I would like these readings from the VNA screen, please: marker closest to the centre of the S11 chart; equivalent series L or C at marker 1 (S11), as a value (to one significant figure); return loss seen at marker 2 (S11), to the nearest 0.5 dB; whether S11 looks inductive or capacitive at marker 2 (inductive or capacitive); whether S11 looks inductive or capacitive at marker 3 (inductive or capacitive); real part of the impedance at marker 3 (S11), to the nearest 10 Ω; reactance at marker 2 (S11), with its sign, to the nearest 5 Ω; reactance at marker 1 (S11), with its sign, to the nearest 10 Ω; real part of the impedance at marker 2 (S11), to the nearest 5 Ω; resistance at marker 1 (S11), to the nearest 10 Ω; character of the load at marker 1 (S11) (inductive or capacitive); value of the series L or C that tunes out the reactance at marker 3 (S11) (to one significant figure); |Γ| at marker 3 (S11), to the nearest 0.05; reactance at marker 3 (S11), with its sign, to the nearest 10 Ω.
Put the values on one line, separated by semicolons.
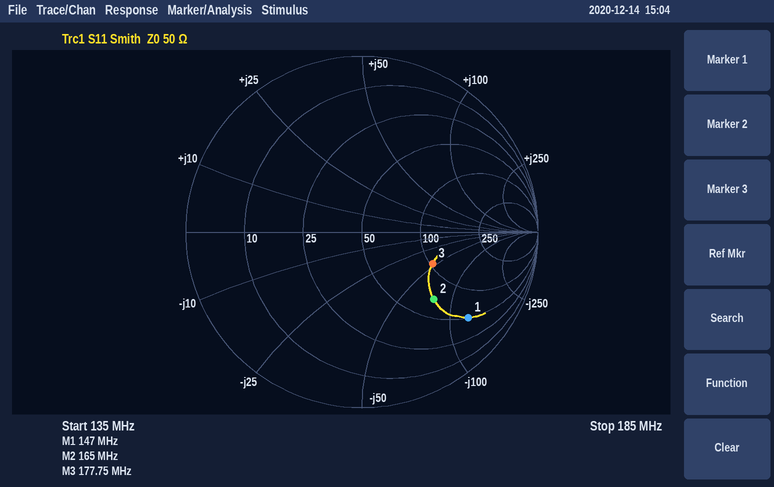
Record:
marker 3; 9 pF; 5.0 dB; capacitive; capacitive; 100 Ω; -75 Ω; -120 Ω; 70 Ω; 50 Ω; capacitive; 40 nH; 0.45; -50 Ω
